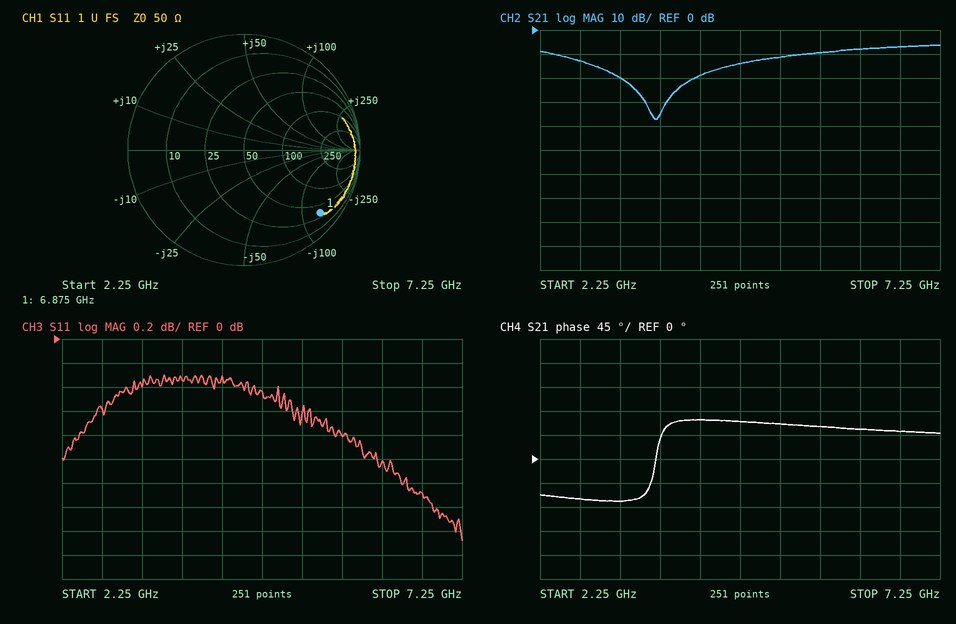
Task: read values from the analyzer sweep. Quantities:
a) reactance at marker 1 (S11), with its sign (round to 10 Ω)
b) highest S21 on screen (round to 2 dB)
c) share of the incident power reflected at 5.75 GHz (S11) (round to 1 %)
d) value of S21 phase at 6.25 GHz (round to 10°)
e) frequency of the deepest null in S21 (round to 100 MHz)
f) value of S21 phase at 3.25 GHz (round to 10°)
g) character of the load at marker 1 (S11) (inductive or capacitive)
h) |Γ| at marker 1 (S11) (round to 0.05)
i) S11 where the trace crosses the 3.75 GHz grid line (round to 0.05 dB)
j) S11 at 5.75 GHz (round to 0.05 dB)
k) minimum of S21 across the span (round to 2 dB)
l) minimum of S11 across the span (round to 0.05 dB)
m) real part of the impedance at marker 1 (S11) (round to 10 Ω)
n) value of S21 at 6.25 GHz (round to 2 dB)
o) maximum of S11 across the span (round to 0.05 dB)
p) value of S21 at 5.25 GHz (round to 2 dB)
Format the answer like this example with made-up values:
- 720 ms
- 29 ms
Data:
- -130 Ω
- -6 dB
- 83 %
- 60°
- 3.7 GHz
- -80°
- capacitive
- 0.85
- -0.35 dB
- -0.80 dB
- -38 dB
- -1.70 dB
- 30 Ω
- -8 dB
- -0.30 dB
- -12 dB
